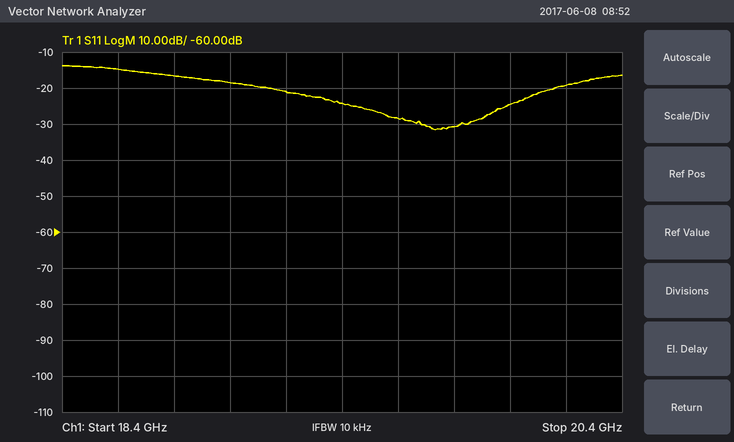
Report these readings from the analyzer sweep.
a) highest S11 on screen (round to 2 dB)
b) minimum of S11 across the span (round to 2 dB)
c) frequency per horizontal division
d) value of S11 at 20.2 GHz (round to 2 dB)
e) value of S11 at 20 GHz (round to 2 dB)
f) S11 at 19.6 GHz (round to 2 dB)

-14 dB
-32 dB
200 MHz
-20 dB
-24 dB
-28 dB
